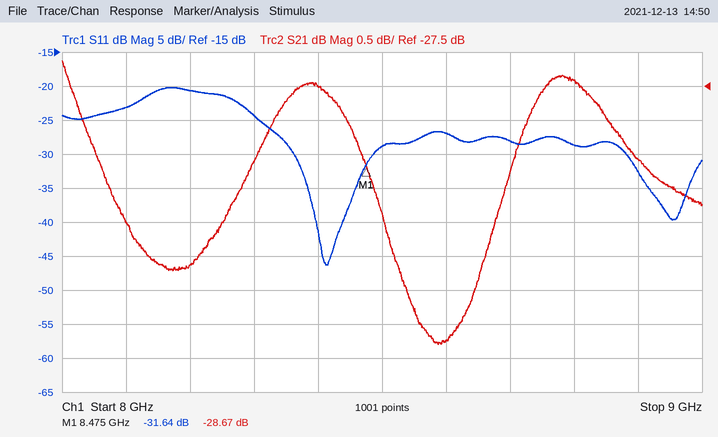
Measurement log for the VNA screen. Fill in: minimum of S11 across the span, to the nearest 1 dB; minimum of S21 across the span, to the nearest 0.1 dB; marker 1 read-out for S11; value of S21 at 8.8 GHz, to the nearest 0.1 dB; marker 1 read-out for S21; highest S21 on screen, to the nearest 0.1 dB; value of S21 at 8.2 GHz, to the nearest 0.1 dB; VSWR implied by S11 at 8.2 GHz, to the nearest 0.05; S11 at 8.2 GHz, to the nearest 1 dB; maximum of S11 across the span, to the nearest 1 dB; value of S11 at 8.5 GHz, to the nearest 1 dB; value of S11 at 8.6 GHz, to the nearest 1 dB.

-46 dB
-31.3 dB
-31.64 dB
-27.4 dB
-28.67 dB
-27.1 dB
-30.1 dB
1.20
-21 dB
-20 dB
-29 dB
-27 dB
